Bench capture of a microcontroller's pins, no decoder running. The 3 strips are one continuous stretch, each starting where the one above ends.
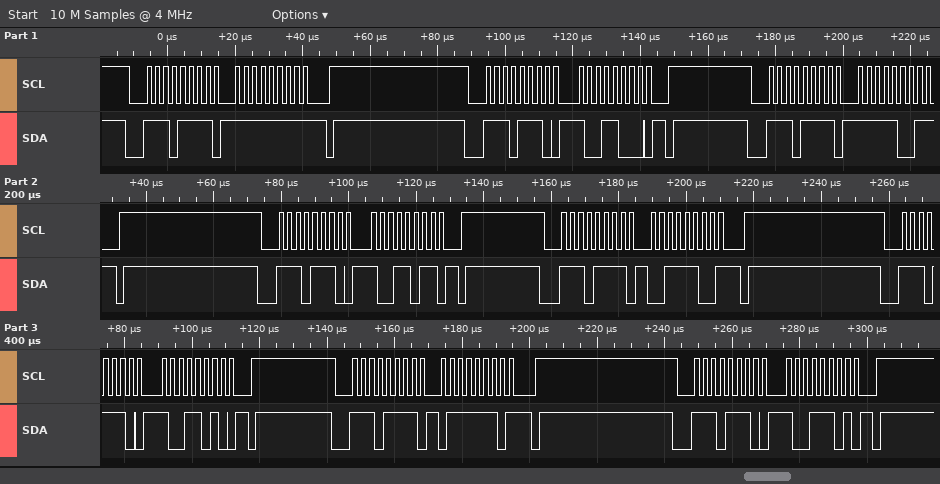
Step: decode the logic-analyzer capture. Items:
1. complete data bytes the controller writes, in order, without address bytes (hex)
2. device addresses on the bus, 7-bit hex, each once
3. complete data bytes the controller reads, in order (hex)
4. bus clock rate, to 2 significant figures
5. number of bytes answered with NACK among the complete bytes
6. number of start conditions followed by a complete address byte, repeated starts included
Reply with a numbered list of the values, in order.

1. 98 9B 9A 9D
2. 0x77
3. FF F9 3C 7E
4. 400 kHz
5. 4
6. 8
